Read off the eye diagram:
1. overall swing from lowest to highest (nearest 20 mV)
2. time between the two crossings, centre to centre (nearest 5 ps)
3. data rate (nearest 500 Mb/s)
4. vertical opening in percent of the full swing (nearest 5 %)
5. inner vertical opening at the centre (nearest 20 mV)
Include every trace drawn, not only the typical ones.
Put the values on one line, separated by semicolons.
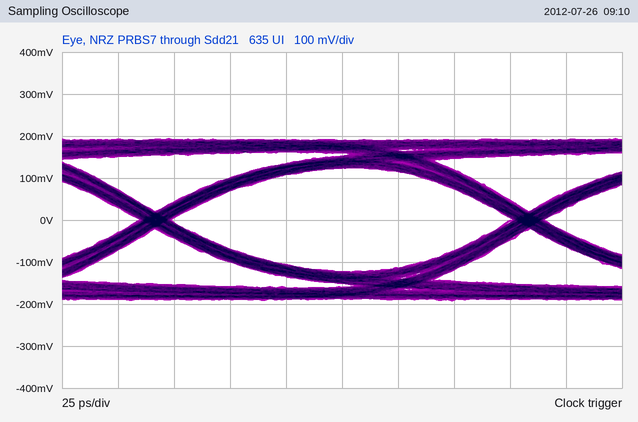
380 mV; 165 ps; 6.0 Gb/s; 65 %; 240 mV
